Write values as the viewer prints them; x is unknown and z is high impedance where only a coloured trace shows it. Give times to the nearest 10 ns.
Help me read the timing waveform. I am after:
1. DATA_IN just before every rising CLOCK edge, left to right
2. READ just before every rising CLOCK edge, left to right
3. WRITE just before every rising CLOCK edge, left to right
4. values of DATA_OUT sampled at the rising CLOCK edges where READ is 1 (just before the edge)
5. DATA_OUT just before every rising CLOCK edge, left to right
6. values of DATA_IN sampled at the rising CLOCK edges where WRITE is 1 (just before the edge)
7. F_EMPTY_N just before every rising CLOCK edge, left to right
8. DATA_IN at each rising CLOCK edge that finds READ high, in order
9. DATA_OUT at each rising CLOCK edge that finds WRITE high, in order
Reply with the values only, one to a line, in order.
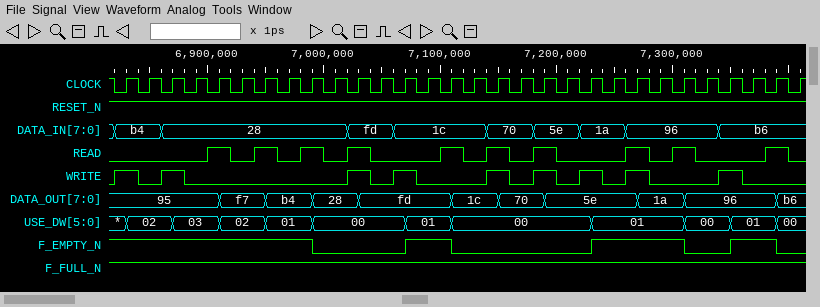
b4, b4, 28, 28, 28, 28, 28, 28, 28, 28, fd, fd, 1c, 1c, 1c, 1c, 70, 70, 5e, 5e, 1a, 1a, 96, 96, 96, 96, b6, b6, b6, b6
0 0 0 0 1 0 1 0 1 0 1 0 0 0 1 0 1 0 1 0 0 0 1 0 1 0 0 0 1 0
1 0 1 0 0 0 0 0 0 0 1 0 1 0 0 0 1 0 1 0 1 0 1 0 0 0 1 0 0 0
95, f7, b4, 28, fd, 1c, 70, 5e, 1a, 96
95, 95, 95, 95, 95, f7, f7, b4, b4, 28, 28, fd, fd, fd, fd, 1c, 1c, 70, 70, 5e, 5e, 5e, 5e, 1a, 1a, 96, 96, 96, 96, b6
b4, 28, fd, 1c, 70, 5e, 1a, 96, b6
1 1 1 1 1 1 1 1 1 0 0 0 0 1 1 0 0 0 0 0 0 1 1 1 1 0 0 1 1 0
28, 28, 28, fd, 1c, 70, 5e, 96, 96, b6
95, 95, 28, fd, 1c, 70, 5e, 5e, 96
